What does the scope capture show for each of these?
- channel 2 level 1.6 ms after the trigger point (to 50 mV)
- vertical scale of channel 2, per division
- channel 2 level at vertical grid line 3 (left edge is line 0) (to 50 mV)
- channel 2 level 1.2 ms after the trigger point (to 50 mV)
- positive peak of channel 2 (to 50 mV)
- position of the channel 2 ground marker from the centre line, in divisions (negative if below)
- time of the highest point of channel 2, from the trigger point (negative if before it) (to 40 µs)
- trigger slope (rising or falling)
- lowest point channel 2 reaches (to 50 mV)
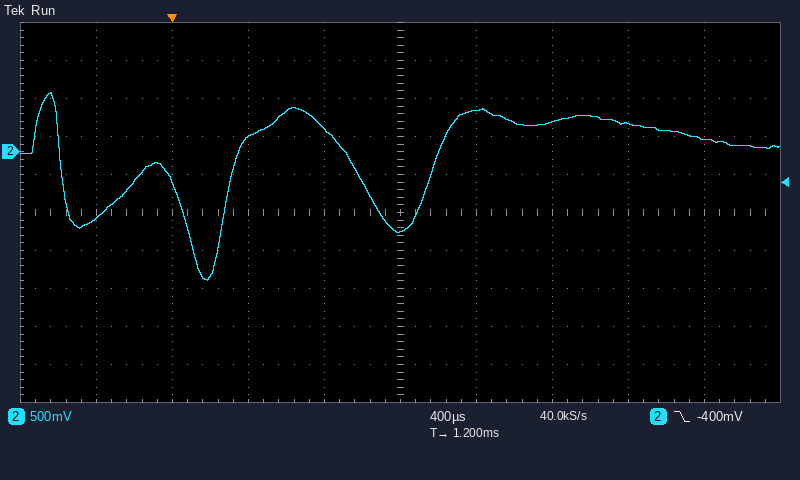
550 mV
500 mV
200 mV
-1.05 V
800 mV
+1.6 div
-640 µs
falling
-1.70 V
